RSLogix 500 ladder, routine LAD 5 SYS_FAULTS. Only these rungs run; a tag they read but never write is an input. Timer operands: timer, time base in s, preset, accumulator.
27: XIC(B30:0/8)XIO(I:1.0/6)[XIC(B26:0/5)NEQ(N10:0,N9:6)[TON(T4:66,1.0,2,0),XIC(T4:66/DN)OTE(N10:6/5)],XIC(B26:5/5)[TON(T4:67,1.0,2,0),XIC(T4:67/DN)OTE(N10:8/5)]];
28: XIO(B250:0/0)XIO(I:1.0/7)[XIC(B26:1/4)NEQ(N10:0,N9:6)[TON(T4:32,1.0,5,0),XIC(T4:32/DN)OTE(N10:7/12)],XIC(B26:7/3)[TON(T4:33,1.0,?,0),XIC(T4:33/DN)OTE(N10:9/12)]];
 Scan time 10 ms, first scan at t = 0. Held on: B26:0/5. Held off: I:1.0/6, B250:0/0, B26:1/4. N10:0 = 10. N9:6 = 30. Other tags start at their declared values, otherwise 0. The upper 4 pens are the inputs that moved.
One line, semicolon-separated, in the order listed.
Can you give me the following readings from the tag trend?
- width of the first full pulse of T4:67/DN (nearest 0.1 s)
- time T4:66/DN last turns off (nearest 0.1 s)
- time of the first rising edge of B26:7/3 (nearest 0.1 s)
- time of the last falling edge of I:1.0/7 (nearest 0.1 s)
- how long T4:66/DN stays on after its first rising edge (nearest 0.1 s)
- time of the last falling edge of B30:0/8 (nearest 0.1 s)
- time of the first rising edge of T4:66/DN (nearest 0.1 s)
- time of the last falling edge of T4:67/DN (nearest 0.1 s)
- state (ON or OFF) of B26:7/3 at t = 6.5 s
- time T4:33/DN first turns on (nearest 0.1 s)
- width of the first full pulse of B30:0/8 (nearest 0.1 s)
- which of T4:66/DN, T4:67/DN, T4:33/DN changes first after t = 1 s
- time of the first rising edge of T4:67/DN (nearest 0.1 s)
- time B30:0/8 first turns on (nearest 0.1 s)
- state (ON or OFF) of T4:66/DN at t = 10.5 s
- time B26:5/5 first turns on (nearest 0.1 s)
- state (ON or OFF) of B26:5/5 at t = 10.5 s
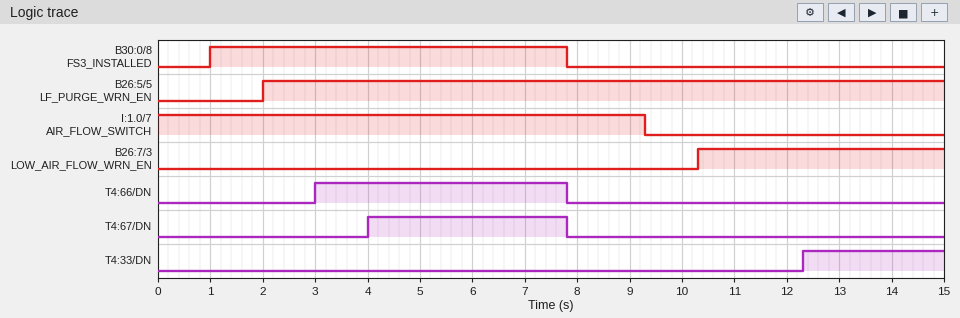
3.8 s; 7.8 s; 10.3 s; 9.3 s; 4.8 s; 7.8 s; 3.0 s; 7.8 s; OFF; 12.3 s; 6.8 s; T4:66/DN; 4.0 s; 1.0 s; OFF; 2.0 s; ON
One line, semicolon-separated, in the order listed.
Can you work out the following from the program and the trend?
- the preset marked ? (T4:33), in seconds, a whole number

2 s
